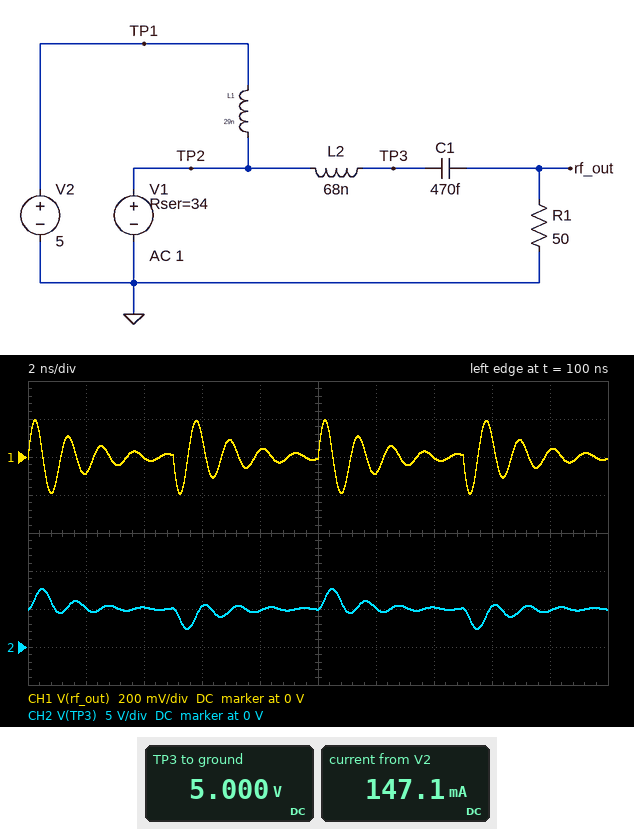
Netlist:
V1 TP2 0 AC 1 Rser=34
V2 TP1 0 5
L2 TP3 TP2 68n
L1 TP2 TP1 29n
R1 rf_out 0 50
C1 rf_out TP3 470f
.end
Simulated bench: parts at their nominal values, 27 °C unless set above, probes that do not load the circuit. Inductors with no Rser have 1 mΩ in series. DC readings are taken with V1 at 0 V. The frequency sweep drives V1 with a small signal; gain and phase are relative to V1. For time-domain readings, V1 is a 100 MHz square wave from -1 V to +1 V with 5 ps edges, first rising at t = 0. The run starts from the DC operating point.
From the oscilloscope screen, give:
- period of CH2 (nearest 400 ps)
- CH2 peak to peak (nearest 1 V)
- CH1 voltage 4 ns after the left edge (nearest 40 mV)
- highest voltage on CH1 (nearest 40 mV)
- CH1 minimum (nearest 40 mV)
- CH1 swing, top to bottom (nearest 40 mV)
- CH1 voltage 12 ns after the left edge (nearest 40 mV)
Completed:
10.0 ns
5 V
0 V
200 mV
-200 mV
400 mV
-80 mV
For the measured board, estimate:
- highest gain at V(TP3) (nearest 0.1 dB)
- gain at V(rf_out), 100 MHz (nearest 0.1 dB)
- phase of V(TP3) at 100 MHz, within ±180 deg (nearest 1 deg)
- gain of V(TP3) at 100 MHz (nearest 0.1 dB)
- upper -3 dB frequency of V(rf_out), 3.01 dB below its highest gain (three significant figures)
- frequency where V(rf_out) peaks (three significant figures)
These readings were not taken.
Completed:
13.3 dB
-43.0 dB
62 deg
-6.4 dB
985 MHz
882 MHz
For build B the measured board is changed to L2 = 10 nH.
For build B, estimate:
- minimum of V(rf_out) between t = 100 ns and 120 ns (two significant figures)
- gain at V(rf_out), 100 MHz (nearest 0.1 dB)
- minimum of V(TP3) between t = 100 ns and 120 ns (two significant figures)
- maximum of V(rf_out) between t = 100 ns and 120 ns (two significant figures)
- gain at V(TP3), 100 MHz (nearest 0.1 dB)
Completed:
-440 mV
-43.1 dB
2.5 V
440 mV
-6.5 dB
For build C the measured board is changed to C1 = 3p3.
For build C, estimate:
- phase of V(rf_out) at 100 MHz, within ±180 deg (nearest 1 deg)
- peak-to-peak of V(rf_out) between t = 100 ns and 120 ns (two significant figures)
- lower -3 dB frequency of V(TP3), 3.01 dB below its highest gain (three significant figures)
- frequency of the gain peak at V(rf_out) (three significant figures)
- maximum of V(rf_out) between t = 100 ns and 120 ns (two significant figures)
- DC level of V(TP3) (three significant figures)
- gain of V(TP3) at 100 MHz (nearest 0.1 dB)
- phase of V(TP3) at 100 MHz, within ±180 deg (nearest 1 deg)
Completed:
144 deg
750 mV
219 MHz
321 MHz
370 mV
5.00 V
-5.5 dB
60 deg
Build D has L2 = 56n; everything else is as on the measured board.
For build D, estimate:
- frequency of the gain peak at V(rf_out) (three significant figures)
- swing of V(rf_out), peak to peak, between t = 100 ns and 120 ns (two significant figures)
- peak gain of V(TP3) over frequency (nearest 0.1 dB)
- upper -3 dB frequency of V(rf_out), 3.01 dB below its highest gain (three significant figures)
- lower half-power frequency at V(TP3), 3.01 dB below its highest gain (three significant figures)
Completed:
972 MHz
410 mV
12.5 dB
1.10 GHz
833 MHz
